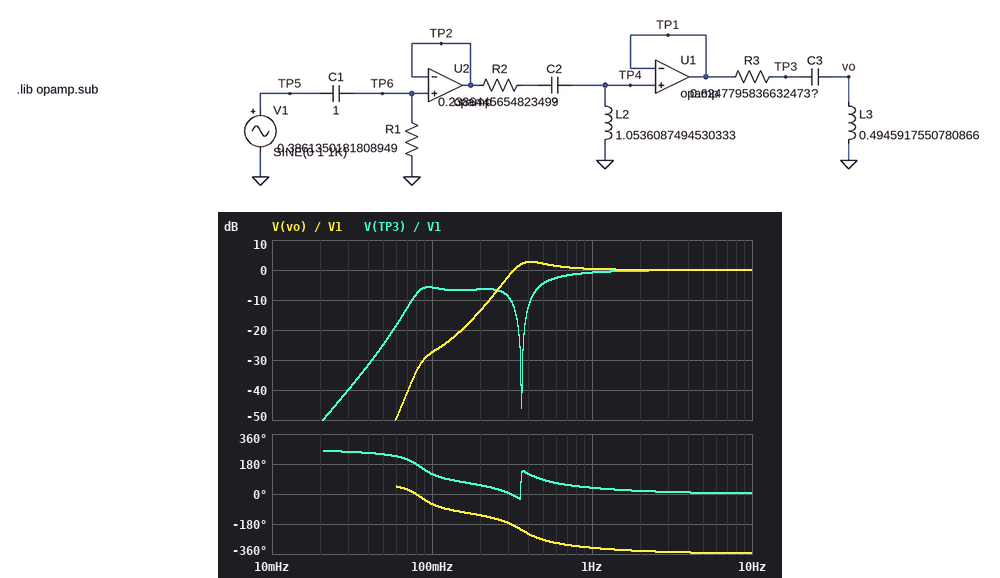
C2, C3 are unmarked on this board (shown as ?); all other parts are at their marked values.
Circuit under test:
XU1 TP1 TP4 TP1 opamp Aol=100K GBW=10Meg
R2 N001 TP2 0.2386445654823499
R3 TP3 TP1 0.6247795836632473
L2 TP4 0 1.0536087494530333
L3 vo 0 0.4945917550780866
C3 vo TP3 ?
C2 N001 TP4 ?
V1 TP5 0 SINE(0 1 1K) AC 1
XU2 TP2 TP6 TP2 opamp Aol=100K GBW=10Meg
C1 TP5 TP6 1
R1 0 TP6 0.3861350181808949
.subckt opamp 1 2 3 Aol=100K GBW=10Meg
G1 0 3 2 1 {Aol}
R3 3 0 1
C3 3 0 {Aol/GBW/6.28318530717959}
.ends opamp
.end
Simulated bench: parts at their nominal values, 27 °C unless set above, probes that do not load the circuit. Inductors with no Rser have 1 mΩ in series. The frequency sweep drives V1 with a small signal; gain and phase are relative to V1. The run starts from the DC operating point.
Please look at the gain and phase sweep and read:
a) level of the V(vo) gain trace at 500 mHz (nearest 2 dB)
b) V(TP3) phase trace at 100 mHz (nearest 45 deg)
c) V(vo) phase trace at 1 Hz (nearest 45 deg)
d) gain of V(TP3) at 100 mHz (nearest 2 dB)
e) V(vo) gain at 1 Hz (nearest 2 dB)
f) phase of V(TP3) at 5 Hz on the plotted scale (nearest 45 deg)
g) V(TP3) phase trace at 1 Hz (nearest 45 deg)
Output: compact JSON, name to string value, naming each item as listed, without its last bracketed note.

{"level of the V(vo) gain trace at 500 mHz": "2 dB", "V(TP3) phase trace at 100 mHz": "135 deg", "V(vo) phase trace at 1 Hz": "-315 deg", "gain of V(TP3) at 100 mHz": "-6 dB", "V(vo) gain at 1 Hz": "0 dB", "phase of V(TP3) at 5 Hz on the plotted scale": "0 deg", "V(TP3) phase trace at 1 Hz": "45 deg"}
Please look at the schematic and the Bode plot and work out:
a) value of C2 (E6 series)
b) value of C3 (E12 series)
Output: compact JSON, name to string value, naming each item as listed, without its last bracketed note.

{"value of C2": "3.3 F", "value of C3": "390 mF"}
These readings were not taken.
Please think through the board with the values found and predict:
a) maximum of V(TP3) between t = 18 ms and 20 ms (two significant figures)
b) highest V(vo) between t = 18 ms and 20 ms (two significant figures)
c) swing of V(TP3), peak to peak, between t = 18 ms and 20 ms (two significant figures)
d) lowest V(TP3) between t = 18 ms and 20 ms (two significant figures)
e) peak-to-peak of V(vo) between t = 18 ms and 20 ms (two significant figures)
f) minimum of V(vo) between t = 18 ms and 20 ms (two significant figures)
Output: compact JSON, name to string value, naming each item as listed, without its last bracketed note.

{"maximum of V(TP3) between t = 18 ms and 20 ms": "1.0 V", "highest V(vo) between t = 18 ms and 20 ms": "1.0 V", "swing of V(TP3), peak to peak, between t = 18 ms and 20 ms": "2.0 V", "lowest V(TP3) between t = 18 ms and 20 ms": "-1.0 V", "peak-to-peak of V(vo) between t = 18 ms and 20 ms": "2.0 V", "minimum of V(vo) between t = 18 ms and 20 ms": "-1.0 V"}
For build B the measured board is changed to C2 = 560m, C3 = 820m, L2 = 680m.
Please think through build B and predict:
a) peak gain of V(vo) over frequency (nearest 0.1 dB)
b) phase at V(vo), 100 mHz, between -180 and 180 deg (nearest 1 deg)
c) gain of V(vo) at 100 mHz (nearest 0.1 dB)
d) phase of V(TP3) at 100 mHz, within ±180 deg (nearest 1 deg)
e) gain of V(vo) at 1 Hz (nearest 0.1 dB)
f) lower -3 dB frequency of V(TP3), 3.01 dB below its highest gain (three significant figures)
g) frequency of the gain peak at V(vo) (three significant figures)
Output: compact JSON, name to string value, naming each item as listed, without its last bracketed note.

{"peak gain of V(vo) over frequency": "10.2 dB", "phase at V(vo), 100 mHz, between -180 and 180 deg": "49 deg", "gain of V(vo) at 100 mHz": "-42.6 dB", "phase of V(TP3) at 100 mHz, within ±180 deg": "-130 deg", "gain of V(vo) at 1 Hz": "0.3 dB", "lower -3 dB frequency of V(TP3), 3.01 dB below its highest gain": "291 mHz", "frequency of the gain peak at V(vo)": "266 mHz"}
